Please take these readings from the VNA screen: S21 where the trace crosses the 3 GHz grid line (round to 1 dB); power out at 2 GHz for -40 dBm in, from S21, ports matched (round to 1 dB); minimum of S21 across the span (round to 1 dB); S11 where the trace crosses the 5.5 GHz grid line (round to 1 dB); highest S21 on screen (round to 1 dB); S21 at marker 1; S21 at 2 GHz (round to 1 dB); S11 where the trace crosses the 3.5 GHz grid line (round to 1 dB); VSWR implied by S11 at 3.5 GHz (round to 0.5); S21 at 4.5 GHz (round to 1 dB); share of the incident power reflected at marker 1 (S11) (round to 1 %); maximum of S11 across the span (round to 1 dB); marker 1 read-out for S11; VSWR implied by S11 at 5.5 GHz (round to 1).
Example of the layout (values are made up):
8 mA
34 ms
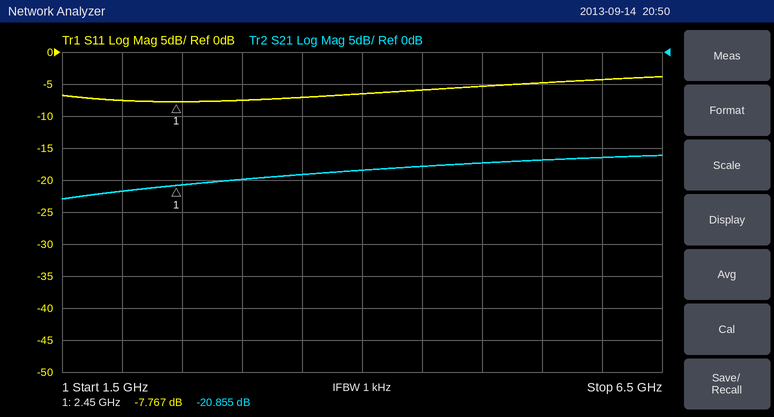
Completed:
-20 dB
-62 dBm
-23 dB
-5 dB
-16 dB
-20.855 dB
-22 dB
-7 dB
2.5
-18 dB
17 %
-4 dB
-7.767 dB
4
